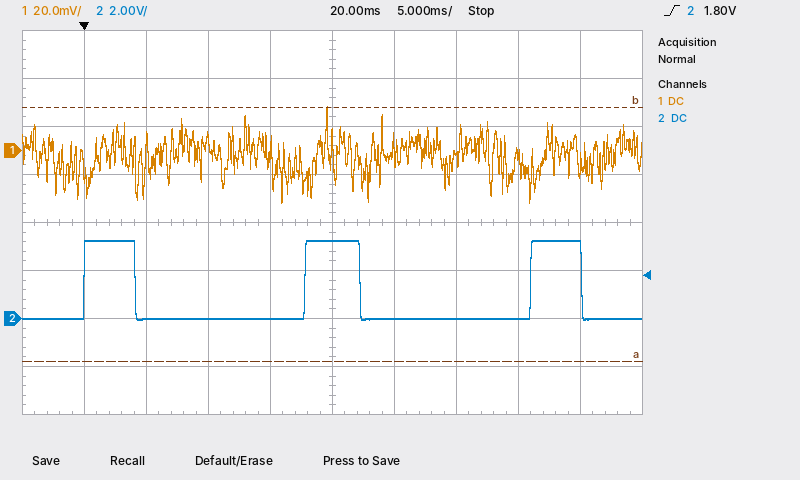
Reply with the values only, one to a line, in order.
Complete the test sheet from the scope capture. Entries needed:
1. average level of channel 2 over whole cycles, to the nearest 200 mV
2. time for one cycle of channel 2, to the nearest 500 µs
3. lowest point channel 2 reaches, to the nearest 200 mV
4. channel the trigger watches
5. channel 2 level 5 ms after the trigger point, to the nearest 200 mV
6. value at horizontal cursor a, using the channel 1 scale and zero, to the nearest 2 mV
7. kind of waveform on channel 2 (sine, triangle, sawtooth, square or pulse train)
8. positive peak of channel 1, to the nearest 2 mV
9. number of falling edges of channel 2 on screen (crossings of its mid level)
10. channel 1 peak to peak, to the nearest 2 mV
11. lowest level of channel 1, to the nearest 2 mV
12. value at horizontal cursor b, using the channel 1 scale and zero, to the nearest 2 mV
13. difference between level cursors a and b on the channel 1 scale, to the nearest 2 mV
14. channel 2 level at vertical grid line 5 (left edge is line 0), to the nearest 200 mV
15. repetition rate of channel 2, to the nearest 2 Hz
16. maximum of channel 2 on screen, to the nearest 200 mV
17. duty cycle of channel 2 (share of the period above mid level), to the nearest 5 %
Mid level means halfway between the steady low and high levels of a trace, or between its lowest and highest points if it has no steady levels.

800 mV
18.0 ms
0.0 V
channel 2
0.0 V
-88 mV
pulse train
18 mV
3
40 mV
-22 mV
18 mV
106 mV
3.2 V
56 Hz
3.2 V
25 %
